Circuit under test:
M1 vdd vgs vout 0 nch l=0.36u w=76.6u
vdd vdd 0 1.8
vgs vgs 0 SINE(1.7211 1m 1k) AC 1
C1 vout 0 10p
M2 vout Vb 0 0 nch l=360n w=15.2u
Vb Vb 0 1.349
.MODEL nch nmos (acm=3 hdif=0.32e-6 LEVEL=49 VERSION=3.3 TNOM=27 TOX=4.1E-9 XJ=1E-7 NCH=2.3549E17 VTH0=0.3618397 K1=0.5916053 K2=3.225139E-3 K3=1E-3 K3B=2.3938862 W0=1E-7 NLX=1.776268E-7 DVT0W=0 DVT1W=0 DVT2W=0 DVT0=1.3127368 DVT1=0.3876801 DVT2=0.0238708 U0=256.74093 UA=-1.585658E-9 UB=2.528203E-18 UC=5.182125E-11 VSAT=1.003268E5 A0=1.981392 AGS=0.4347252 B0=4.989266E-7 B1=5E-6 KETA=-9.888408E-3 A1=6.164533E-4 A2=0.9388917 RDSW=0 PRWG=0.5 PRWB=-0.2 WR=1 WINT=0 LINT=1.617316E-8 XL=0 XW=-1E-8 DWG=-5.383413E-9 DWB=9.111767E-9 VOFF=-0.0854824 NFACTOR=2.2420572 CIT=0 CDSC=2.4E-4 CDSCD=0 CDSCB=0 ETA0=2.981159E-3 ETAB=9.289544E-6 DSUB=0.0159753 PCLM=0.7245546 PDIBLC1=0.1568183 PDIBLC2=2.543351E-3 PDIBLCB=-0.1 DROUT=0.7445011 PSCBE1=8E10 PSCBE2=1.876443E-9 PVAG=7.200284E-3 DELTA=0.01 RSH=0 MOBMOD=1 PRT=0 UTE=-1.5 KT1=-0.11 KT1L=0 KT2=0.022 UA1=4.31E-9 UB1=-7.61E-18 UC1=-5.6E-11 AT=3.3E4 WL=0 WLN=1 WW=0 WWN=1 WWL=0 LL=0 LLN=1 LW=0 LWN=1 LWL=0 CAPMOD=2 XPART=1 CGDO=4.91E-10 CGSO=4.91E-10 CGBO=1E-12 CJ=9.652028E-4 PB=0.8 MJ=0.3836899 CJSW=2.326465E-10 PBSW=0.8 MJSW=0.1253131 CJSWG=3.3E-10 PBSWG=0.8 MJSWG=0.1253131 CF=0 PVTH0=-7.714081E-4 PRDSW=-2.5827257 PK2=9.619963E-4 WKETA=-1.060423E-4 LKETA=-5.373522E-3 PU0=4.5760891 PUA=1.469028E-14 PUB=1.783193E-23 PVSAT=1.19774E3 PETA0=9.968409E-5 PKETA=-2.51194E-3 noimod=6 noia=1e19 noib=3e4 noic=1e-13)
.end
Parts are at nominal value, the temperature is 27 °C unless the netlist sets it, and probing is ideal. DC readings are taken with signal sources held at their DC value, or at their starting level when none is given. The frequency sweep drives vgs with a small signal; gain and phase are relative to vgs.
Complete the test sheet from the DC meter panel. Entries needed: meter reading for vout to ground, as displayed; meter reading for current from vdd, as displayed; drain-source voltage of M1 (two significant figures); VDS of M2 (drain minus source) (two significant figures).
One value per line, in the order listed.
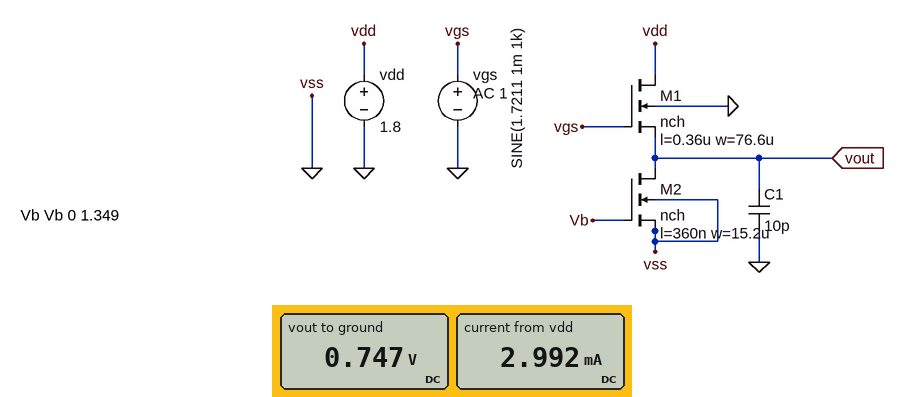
0.747 V
2.992 mA
1.1 V
750 mV
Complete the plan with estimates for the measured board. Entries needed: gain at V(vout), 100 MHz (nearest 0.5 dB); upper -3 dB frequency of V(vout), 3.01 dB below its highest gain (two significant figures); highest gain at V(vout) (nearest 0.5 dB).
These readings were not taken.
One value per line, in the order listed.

-2.5 dB
310 MHz
-2.0 dB
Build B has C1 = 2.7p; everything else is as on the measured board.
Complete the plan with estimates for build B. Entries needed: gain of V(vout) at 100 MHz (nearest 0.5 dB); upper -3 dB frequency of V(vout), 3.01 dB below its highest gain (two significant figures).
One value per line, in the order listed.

-2.0 dB
1.1 GHz
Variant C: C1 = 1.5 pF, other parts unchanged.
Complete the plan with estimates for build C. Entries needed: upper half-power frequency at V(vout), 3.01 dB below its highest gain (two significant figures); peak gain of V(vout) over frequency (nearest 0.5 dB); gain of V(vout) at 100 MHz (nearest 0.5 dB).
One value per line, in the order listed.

1.8 GHz
-2.0 dB
-2.0 dB
